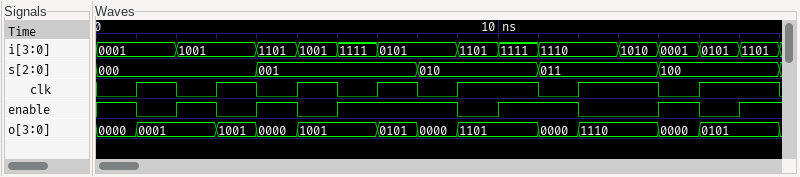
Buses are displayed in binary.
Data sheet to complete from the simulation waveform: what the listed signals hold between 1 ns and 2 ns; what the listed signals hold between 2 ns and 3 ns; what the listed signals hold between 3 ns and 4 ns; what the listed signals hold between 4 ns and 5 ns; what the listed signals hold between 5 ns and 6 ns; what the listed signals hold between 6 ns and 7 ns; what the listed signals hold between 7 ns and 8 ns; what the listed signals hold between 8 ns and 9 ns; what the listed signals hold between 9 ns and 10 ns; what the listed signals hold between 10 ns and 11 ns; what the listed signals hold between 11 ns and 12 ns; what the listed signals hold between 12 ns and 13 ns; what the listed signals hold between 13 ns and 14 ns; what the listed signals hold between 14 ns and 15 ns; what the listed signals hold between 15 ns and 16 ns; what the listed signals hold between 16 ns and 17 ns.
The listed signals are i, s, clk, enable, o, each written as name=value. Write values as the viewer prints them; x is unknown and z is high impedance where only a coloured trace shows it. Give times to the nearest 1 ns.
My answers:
i=0001, s=000, clk=1, enable=0, o=0001
i=1001, s=000, clk=0, enable=1, o=0001
i=1001, s=000, clk=1, enable=0, o=1001
i=1101, s=001, clk=0, enable=1, o=0000
i=1001, s=001, clk=1, enable=0, o=1001
i=1111, s=001, clk=0, enable=1, o=1001
i=0101, s=001, clk=1, enable=1, o=0101
i=0101, s=010, clk=0, enable=1, o=0000
i=1101, s=010, clk=1, enable=0, o=1101
i=1111, s=010, clk=1, enable=1, o=1101
i=1110, s=011, clk=0, enable=1, o=0000
i=1110, s=011, clk=1, enable=0, o=1110
i=1010, s=011, clk=1, enable=0, o=1110
i=0001, s=100, clk=0, enable=1, o=0000
i=0101, s=100, clk=1, enable=0, o=0101
i=1101, s=100, clk=1, enable=1, o=0101
